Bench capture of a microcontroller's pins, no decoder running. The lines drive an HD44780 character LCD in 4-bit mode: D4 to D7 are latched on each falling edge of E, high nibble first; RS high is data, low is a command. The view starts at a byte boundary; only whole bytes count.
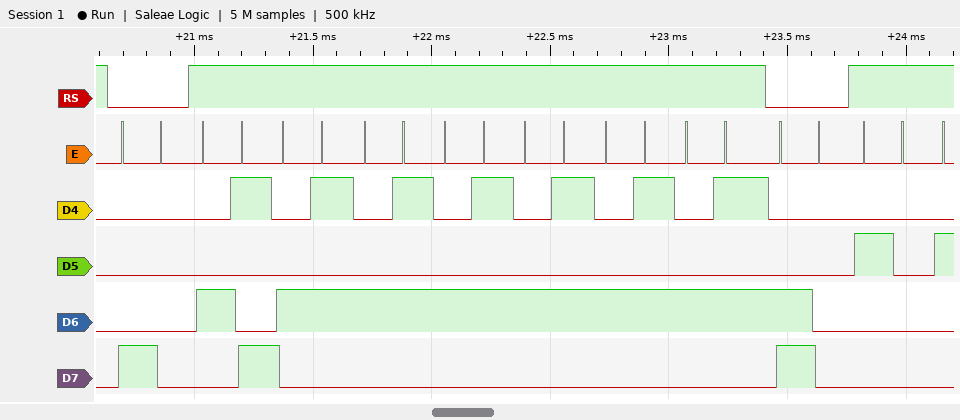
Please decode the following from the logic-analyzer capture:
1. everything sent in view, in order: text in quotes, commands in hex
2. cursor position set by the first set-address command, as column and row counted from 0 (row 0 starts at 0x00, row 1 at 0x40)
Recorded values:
0x80 "IEEEEEE" 0xC0 " "
column 0, row 0
